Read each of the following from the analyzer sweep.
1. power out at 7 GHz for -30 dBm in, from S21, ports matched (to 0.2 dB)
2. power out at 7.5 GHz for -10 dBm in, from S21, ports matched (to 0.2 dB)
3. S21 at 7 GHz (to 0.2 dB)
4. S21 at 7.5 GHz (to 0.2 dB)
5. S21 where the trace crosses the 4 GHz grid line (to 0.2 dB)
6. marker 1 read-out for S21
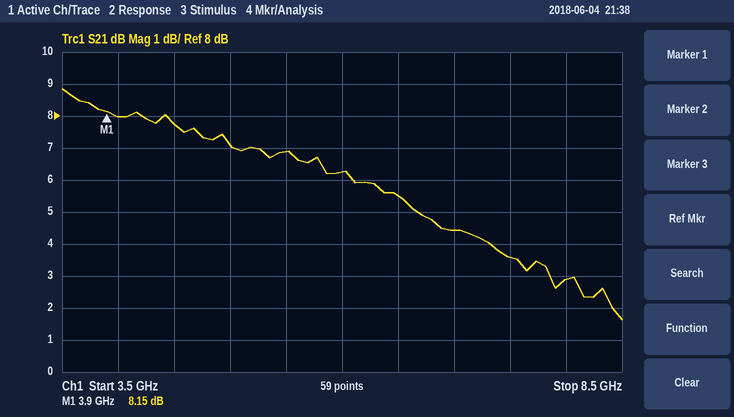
-25.6 dBm
-6.4 dBm
4.4 dB
3.6 dB
8.0 dB
8.15 dB
